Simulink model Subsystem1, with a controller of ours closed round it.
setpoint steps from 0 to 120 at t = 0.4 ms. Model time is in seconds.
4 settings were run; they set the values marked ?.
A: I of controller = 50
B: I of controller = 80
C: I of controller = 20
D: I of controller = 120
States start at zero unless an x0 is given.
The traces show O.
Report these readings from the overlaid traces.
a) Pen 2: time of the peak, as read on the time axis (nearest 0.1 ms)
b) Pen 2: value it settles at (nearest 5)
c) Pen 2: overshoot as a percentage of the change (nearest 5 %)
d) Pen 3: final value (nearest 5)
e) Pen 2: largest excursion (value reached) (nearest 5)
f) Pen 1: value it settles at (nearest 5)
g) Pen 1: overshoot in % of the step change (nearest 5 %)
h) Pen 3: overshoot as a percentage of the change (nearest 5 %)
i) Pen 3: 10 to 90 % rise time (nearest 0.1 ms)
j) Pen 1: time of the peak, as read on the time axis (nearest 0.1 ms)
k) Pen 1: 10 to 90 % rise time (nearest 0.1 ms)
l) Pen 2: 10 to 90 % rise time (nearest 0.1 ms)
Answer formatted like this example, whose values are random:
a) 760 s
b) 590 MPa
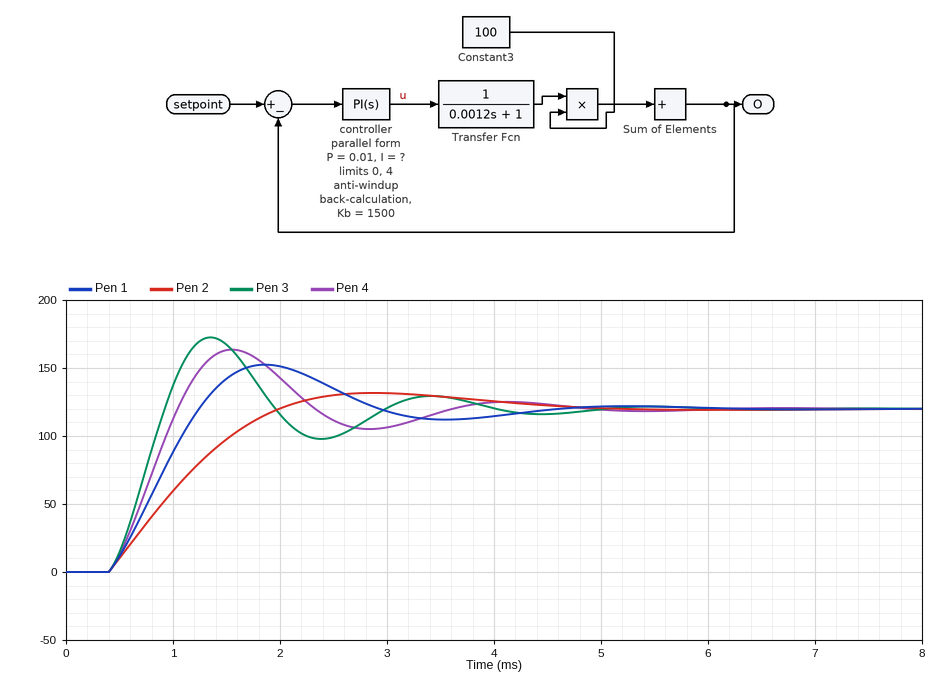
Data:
a) 2.9 ms
b) 120
c) 10 %
d) 120
e) 130
f) 120
g) 25 %
h) 45 %
i) 0.4 ms
j) 1.9 ms
k) 0.6 ms
l) 1.2 ms
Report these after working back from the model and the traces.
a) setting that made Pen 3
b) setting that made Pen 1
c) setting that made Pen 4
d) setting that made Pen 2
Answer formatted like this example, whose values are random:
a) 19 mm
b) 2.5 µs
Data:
a) D
b) A
c) B
d) C
